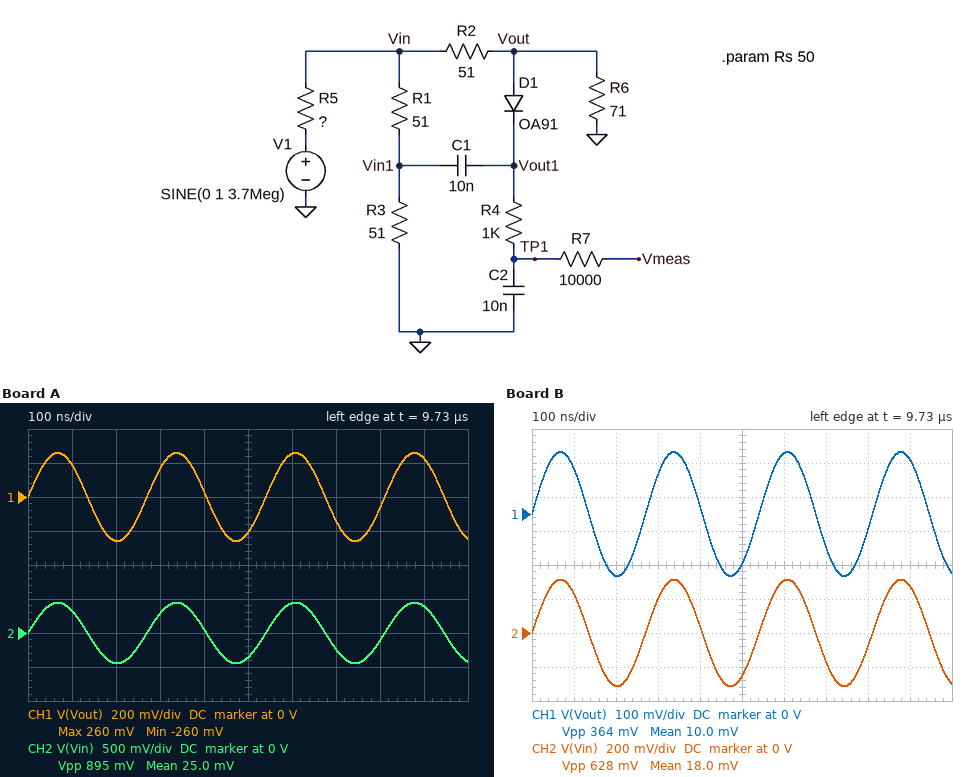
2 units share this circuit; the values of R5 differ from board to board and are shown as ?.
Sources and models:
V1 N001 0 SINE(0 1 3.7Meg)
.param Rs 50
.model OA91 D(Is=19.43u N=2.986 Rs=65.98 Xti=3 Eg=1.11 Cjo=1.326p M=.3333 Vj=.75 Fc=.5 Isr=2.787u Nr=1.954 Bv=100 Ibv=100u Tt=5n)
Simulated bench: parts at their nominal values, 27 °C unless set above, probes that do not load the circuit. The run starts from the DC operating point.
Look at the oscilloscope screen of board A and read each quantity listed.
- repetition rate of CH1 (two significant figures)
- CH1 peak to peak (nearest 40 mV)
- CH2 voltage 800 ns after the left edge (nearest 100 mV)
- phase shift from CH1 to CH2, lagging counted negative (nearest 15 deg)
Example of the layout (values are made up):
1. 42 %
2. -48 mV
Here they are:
1. 3.7 MHz
2. 520 mV
3. -100 mV
4. 0 deg
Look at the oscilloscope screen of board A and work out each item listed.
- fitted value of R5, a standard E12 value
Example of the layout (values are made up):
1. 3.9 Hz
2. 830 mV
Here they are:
1. 68 Ω
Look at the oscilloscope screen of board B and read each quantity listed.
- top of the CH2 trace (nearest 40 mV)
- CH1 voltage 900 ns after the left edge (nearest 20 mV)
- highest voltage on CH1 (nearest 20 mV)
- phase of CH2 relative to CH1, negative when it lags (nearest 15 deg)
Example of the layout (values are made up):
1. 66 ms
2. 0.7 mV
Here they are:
1. 320 mV
2. 160 mV
3. 180 mV
4. 0 deg
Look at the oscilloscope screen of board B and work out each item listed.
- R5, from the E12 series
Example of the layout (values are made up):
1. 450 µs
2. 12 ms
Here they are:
1. 120 Ω
